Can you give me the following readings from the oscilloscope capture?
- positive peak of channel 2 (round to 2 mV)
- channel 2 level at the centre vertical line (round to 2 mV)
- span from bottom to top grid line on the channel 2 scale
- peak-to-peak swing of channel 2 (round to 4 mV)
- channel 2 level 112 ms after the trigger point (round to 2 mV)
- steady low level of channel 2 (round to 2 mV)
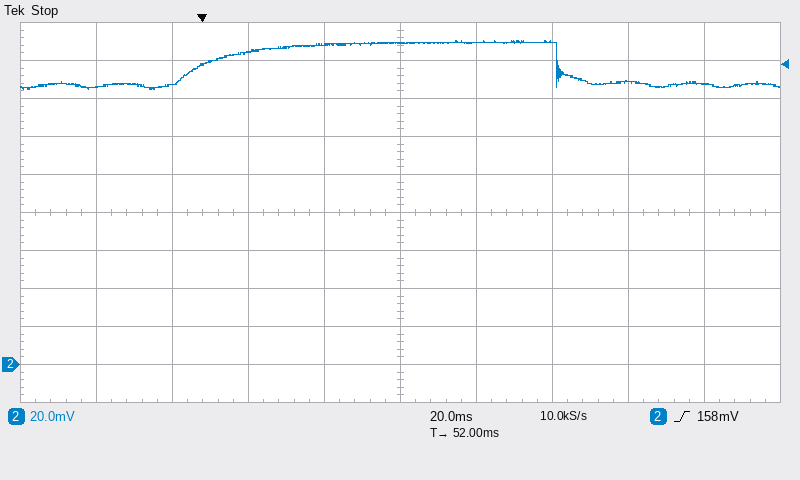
170 mV
170 mV
200 mV
24 mV
148 mV
148 mV
